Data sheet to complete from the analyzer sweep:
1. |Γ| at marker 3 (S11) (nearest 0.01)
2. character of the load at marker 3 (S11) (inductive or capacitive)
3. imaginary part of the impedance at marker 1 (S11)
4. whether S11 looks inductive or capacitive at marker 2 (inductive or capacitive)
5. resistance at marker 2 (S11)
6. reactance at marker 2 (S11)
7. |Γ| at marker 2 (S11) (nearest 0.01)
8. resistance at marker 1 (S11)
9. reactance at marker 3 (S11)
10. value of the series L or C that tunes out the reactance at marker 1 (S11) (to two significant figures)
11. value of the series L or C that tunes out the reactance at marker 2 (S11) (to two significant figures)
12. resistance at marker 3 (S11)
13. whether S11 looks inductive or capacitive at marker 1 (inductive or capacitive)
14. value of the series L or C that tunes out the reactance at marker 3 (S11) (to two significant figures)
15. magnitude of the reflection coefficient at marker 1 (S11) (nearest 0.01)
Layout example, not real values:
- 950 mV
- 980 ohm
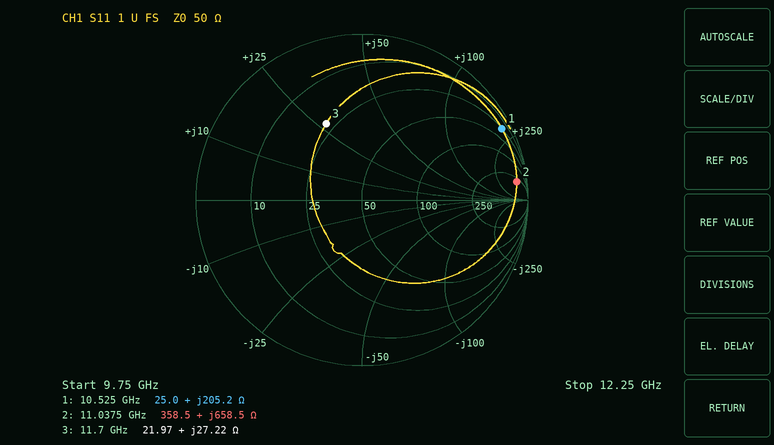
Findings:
- 0.51
- inductive
- +205.2 Ω
- inductive
- 358.5 Ω
- +658.5 Ω
- 0.94
- 25.0 Ω
- +27.22 Ω
- 74 fF
- 22 fF
- 21.97 Ω
- inductive
- 500 fF
- 0.95
